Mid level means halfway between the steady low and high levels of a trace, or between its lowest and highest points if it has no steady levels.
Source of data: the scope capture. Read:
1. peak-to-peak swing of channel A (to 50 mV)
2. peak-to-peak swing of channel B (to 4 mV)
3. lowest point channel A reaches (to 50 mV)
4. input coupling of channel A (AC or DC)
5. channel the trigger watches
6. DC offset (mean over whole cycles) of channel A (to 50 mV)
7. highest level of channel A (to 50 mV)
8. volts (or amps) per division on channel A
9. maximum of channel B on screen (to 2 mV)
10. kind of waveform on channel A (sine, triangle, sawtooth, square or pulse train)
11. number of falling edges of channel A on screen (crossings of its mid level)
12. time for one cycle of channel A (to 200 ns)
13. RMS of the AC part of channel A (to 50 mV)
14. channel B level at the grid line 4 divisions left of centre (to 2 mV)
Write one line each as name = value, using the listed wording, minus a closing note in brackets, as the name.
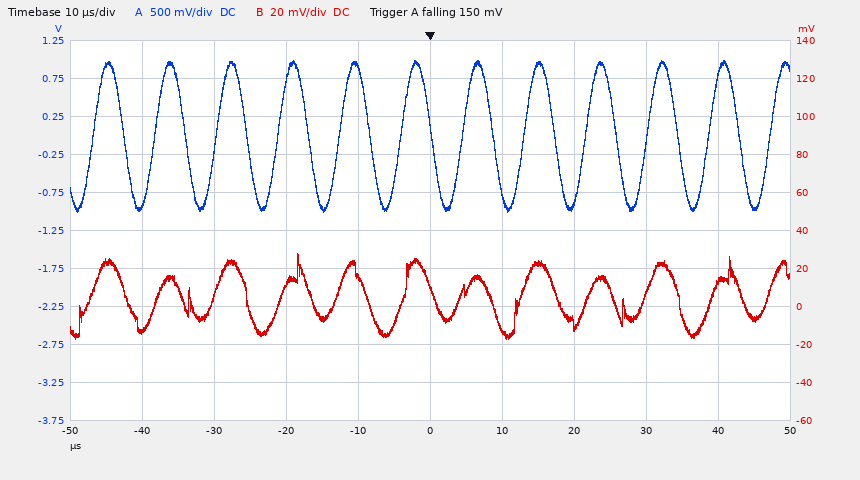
peak-to-peak swing of channel A = 2.00 V
peak-to-peak swing of channel B = 44 mV
lowest point channel A reaches = -1.00 V
input coupling of channel A = DC
channel the trigger watches = channel A
DC offset (mean over whole cycles) of channel A = 0 mV
highest level of channel A = 1.00 V
volts (or amps) per division on channel A = 500 mV
maximum of channel B on screen = 28 mV
kind of waveform on channel A = sine
number of falling edges of channel A on screen = 11
time for one cycle of channel A = 8.6 µs
RMS of the AC part of channel A = 700 mV
channel B level at the grid line 4 divisions left of centre = -12 mV
